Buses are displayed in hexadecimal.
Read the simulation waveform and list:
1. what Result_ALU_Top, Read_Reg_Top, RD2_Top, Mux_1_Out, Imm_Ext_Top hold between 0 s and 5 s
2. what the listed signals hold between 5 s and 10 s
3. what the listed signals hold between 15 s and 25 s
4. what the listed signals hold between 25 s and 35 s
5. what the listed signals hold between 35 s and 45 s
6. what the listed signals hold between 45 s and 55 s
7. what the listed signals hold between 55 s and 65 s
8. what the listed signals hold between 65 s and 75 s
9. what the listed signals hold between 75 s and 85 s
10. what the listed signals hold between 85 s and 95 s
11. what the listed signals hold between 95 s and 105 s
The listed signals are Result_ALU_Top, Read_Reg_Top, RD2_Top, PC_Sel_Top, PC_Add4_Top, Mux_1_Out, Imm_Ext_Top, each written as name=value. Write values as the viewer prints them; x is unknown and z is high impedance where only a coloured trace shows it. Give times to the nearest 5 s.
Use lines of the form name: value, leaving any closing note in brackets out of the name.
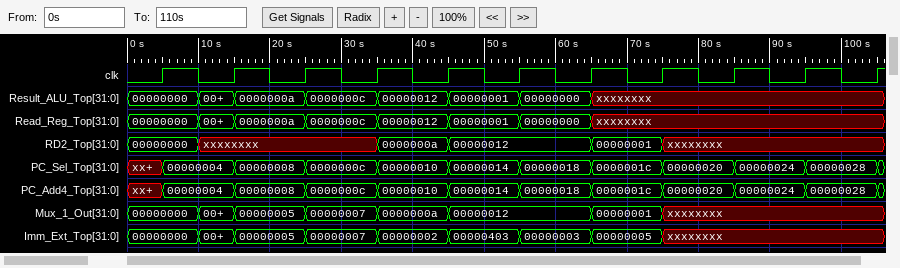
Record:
what Result_ALU_Top, Read_Reg_Top, RD2_Top, Mux_1_Out, Imm_Ext_Top hold between 0 s and 5 s: Result_ALU_Top=00000000, Read_Reg_Top=00000000, RD2_Top=00000000, Mux_1_Out=00000000, Imm_Ext_Top=00000000
what the listed signals hold between 5 s and 10 s: Result_ALU_Top=00000000, Read_Reg_Top=00000000, RD2_Top=00000000, PC_Sel_Top=00000004, PC_Add4_Top=00000004, Mux_1_Out=00000000, Imm_Ext_Top=00000000
what the listed signals hold between 15 s and 25 s: Result_ALU_Top=0000000a, Read_Reg_Top=0000000a, RD2_Top=xxxxxxxx, PC_Sel_Top=00000008, PC_Add4_Top=00000008, Mux_1_Out=00000005, Imm_Ext_Top=00000005
what the listed signals hold between 25 s and 35 s: Result_ALU_Top=0000000c, Read_Reg_Top=0000000c, RD2_Top=xxxxxxxx, PC_Sel_Top=0000000c, PC_Add4_Top=0000000c, Mux_1_Out=00000007, Imm_Ext_Top=00000007
what the listed signals hold between 35 s and 45 s: Result_ALU_Top=00000012, Read_Reg_Top=00000012, RD2_Top=0000000a, PC_Sel_Top=00000010, PC_Add4_Top=00000010, Mux_1_Out=0000000a, Imm_Ext_Top=00000002
what the listed signals hold between 45 s and 55 s: Result_ALU_Top=00000001, Read_Reg_Top=00000001, RD2_Top=00000012, PC_Sel_Top=00000014, PC_Add4_Top=00000014, Mux_1_Out=00000012, Imm_Ext_Top=00000403
what the listed signals hold between 55 s and 65 s: Result_ALU_Top=00000000, Read_Reg_Top=00000000, RD2_Top=00000012, PC_Sel_Top=00000018, PC_Add4_Top=00000018, Mux_1_Out=00000012, Imm_Ext_Top=00000003
what the listed signals hold between 65 s and 75 s: Result_ALU_Top=xxxxxxxx, Read_Reg_Top=xxxxxxxx, RD2_Top=00000001, PC_Sel_Top=0000001c, PC_Add4_Top=0000001c, Mux_1_Out=00000001, Imm_Ext_Top=00000005
what the listed signals hold between 75 s and 85 s: Result_ALU_Top=xxxxxxxx, Read_Reg_Top=xxxxxxxx, RD2_Top=xxxxxxxx, PC_Sel_Top=00000020, PC_Add4_Top=00000020, Mux_1_Out=xxxxxxxx, Imm_Ext_Top=xxxxxxxx
what the listed signals hold between 85 s and 95 s: Result_ALU_Top=xxxxxxxx, Read_Reg_Top=xxxxxxxx, RD2_Top=xxxxxxxx, PC_Sel_Top=00000024, PC_Add4_Top=00000024, Mux_1_Out=xxxxxxxx, Imm_Ext_Top=xxxxxxxx
what the listed signals hold between 95 s and 105 s: Result_ALU_Top=xxxxxxxx, Read_Reg_Top=xxxxxxxx, RD2_Top=xxxxxxxx, PC_Sel_Top=00000028, PC_Add4_Top=00000028, Mux_1_Out=xxxxxxxx, Imm_Ext_Top=xxxxxxxx
